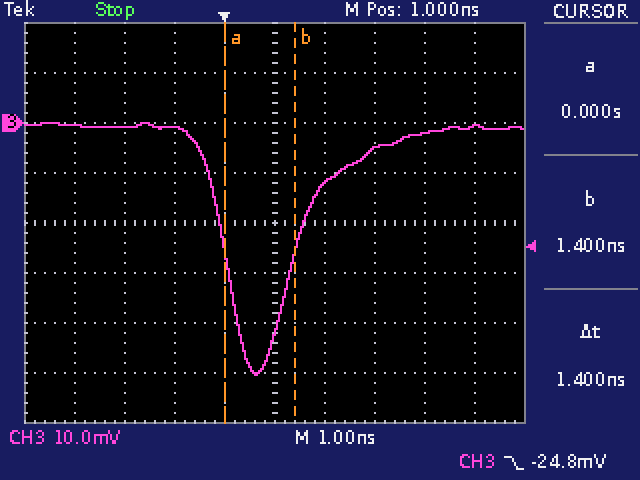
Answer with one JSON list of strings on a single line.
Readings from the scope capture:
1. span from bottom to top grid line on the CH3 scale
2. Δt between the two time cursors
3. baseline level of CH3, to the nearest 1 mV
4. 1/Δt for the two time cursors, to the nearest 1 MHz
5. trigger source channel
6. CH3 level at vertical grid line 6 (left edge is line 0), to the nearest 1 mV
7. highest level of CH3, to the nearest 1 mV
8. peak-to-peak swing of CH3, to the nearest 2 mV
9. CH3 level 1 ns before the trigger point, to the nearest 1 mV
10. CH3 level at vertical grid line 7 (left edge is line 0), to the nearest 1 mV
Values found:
["80 mV", "1.4 ns", "-1 mV", "714 MHz", "CH3", "-12 mV", "0 mV", "50 mV", "-1 mV", "-5 mV"]
